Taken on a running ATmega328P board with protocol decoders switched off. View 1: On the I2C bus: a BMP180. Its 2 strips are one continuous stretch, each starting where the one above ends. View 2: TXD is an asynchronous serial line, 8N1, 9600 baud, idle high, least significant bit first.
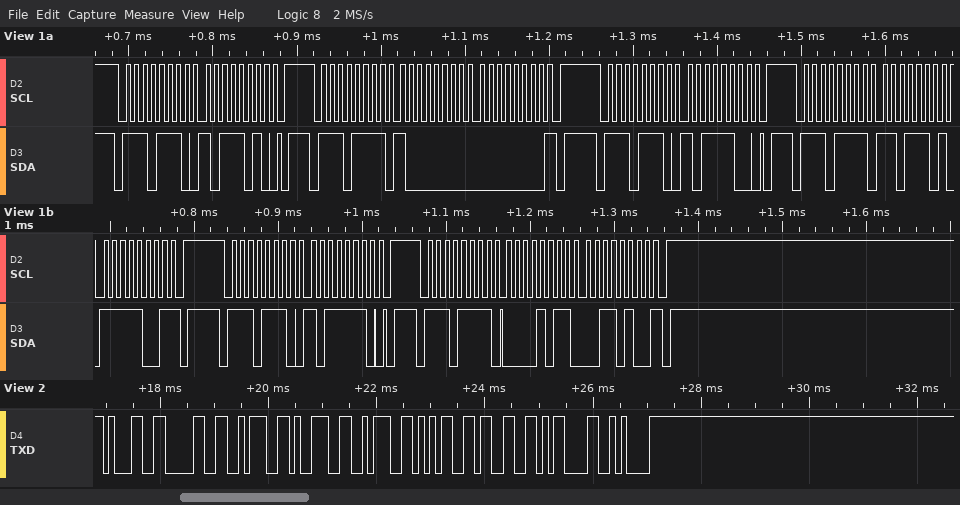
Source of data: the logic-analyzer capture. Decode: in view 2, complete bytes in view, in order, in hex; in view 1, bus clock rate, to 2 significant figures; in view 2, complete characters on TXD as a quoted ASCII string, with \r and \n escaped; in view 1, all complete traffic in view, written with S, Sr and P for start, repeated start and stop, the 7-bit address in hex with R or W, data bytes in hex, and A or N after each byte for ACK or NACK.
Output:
31 30 3A 39 3A 35 33 0D 0A
100 kHz
"10:9:53\r\n"
S 77W A BA A P S 77R A 80 A 00 N P S 77W A BC A P S 77R A DD A F9 N P S 77W A BE A P S 77R A 0B A 34 N P
